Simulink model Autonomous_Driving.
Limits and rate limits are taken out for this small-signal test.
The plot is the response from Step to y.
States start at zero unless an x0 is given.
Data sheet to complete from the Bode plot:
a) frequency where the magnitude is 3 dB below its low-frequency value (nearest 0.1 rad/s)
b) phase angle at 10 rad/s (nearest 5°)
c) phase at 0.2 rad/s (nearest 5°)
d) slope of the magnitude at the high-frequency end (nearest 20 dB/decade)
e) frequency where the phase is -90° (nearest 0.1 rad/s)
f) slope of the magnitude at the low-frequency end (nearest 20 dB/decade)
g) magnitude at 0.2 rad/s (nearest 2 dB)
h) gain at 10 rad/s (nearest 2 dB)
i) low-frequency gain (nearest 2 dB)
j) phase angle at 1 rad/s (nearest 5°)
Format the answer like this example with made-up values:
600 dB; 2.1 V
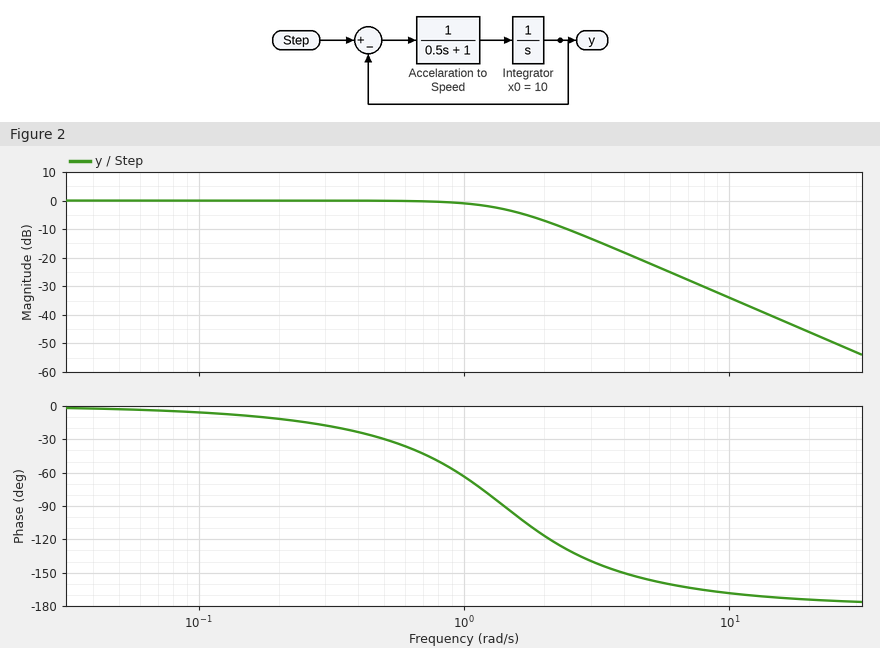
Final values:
1.4 rad/s; -170°; -10°; -40 dB/decade; 1.4 rad/s; 0 dB/decade; 0 dB; -34 dB; 0 dB; -65°
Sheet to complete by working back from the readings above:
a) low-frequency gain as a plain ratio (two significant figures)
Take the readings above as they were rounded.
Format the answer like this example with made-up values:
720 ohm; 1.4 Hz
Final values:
1.0
